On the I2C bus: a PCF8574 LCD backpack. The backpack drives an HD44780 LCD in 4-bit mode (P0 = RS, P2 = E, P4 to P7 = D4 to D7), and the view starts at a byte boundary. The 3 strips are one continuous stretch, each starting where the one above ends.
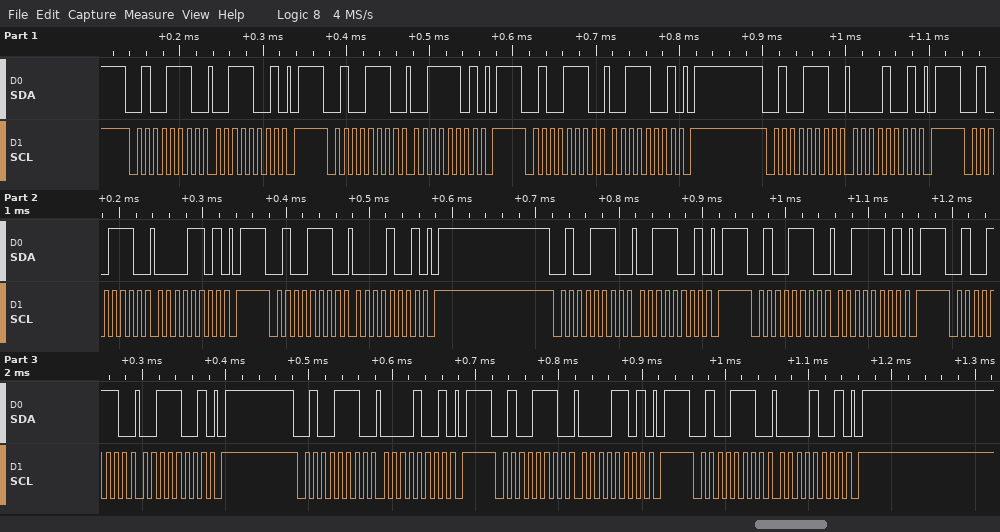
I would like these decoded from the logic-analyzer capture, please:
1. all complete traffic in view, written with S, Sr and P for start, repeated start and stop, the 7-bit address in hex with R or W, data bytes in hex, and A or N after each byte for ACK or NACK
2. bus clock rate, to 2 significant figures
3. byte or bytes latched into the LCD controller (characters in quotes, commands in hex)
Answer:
S 27W A 39 A P S 27W A 3D A P S 27W A 39 A P S 27W A 09 A P S 27W A 0D A P S 27W A 09 A P S 27W A 39 A P S 27W A 3D A P S 27W A 39 A P S 27W A 09 A P S 27W A 0D A P S 27W A 09 A P
100 kHz
'0' '0'
